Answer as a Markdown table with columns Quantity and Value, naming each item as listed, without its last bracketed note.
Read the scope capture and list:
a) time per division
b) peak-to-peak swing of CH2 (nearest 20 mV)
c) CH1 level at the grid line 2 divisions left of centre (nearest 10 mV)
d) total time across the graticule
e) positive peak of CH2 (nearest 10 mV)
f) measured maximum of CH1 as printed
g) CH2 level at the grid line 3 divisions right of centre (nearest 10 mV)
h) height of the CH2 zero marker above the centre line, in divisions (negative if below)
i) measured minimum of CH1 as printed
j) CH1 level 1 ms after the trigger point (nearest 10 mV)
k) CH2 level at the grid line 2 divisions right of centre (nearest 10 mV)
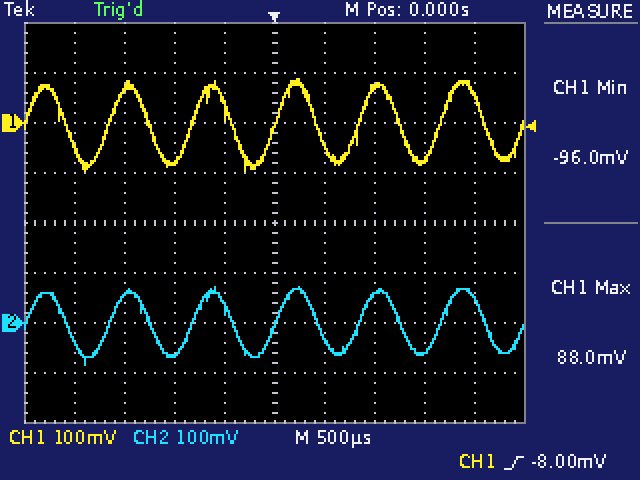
| Quantity | Value |
|---|---|
| time per division | 500 µs |
| peak-to-peak swing of CH2 | 160 mV |
| CH1 level at the grid line 2 divisions left of centre | -80 mV |
| total time across the graticule | 5 ms |
| positive peak of CH2 | 70 mV |
| measured maximum of CH1 as printed | 88.0 mV |
| CH2 level at the grid line 3 divisions right of centre | -60 mV |
| height of the CH2 zero marker above the centre line, in divisions | -2.0 div |
| measured minimum of CH1 as printed | -96.0 mV |
| CH1 level 1 ms after the trigger point | 70 mV |
| CH2 level at the grid line 2 divisions right of centre | 60 mV |
